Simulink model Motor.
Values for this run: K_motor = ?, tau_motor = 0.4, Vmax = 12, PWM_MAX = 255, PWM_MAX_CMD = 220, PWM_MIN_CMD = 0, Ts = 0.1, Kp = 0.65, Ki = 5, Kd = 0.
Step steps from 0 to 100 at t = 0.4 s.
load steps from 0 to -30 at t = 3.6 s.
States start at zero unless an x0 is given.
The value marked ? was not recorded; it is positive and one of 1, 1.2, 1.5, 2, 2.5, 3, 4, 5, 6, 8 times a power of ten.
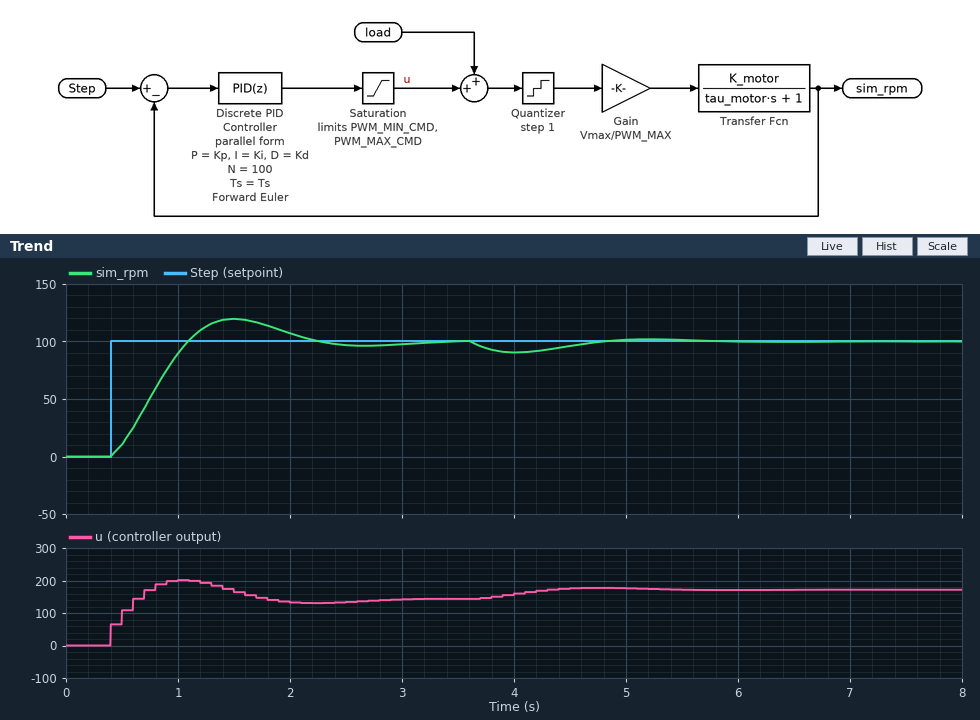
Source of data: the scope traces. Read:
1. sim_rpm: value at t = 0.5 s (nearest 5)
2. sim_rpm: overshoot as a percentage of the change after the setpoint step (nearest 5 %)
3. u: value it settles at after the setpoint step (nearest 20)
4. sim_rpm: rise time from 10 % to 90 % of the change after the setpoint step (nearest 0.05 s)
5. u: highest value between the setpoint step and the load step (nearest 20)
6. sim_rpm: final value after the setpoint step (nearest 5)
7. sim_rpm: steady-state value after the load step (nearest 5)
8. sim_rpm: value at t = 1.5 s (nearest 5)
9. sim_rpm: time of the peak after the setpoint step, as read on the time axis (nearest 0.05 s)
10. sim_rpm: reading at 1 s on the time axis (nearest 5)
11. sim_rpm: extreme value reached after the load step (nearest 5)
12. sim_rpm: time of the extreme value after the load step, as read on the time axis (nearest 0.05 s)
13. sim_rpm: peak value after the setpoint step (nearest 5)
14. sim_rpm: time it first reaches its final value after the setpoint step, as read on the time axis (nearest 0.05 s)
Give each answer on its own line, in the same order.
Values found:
10
20 %
140
0.50 s
200
100
100
120
1.50 s
90
90
4.00 s
120
1.10 s
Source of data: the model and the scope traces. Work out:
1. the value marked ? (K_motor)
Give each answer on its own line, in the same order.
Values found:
15
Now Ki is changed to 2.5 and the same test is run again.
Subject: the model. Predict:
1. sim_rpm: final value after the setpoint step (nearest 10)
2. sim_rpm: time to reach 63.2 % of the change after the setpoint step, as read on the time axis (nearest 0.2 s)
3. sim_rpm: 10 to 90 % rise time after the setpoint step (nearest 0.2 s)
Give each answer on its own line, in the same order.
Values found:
100
1.0 s
1.0 s
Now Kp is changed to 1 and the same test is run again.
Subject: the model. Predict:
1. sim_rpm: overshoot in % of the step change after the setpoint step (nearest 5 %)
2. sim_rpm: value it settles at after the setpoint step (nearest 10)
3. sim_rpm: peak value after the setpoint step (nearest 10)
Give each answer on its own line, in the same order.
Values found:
10 %
100
110
